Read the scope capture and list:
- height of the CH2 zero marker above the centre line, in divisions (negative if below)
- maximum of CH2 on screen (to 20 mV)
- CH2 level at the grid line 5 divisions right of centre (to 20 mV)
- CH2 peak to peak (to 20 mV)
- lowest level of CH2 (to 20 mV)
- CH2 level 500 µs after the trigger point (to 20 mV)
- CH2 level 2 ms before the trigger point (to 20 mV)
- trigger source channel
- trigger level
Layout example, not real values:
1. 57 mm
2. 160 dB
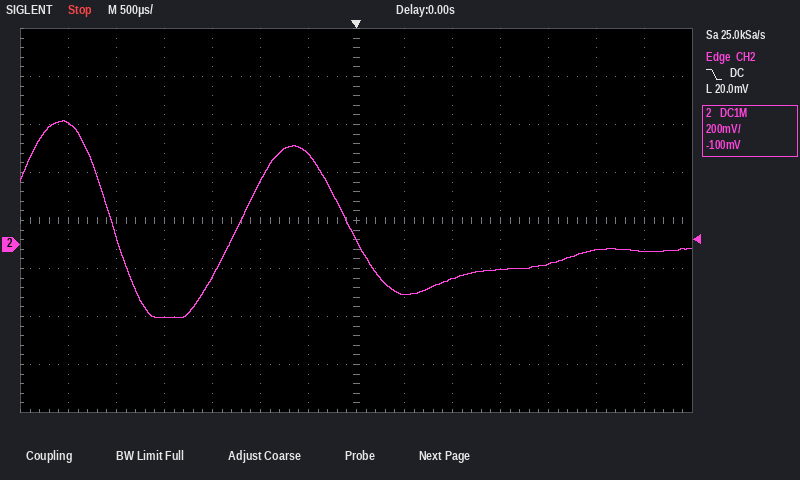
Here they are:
1. -0.5 div
2. 520 mV
3. -20 mV
4. 820 mV
5. -300 mV
6. -200 mV
7. -300 mV
8. CH2
9. 20.0 mV
